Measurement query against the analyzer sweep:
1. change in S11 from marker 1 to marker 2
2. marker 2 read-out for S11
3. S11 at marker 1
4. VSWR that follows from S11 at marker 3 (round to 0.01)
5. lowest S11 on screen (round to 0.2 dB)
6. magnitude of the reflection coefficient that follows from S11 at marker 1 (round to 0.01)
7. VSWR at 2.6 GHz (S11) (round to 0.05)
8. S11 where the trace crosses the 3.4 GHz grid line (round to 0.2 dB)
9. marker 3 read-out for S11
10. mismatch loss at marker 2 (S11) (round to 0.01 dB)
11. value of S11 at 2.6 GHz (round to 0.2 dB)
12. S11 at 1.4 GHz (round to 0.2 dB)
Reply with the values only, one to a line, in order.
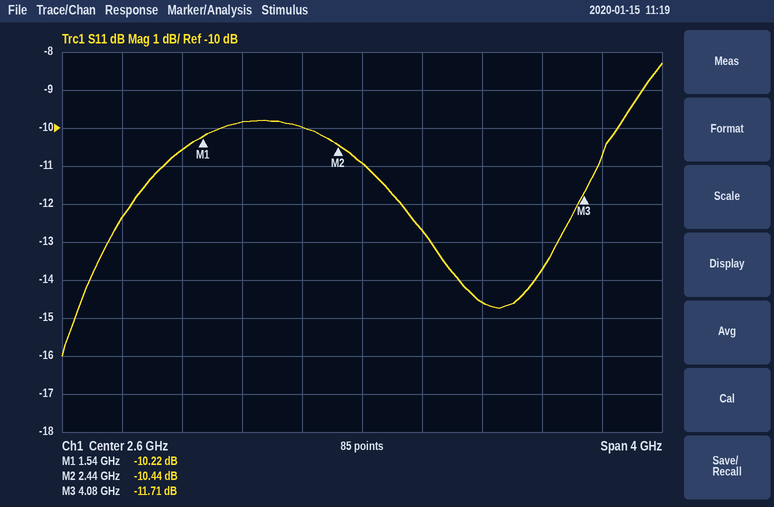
-0.22 dB
-10.44 dB
-10.22 dB
1.70
-16.0 dB
0.31
1.80
-14.6 dB
-11.71 dB
0.41 dB
-11.0 dB
-10.6 dB
